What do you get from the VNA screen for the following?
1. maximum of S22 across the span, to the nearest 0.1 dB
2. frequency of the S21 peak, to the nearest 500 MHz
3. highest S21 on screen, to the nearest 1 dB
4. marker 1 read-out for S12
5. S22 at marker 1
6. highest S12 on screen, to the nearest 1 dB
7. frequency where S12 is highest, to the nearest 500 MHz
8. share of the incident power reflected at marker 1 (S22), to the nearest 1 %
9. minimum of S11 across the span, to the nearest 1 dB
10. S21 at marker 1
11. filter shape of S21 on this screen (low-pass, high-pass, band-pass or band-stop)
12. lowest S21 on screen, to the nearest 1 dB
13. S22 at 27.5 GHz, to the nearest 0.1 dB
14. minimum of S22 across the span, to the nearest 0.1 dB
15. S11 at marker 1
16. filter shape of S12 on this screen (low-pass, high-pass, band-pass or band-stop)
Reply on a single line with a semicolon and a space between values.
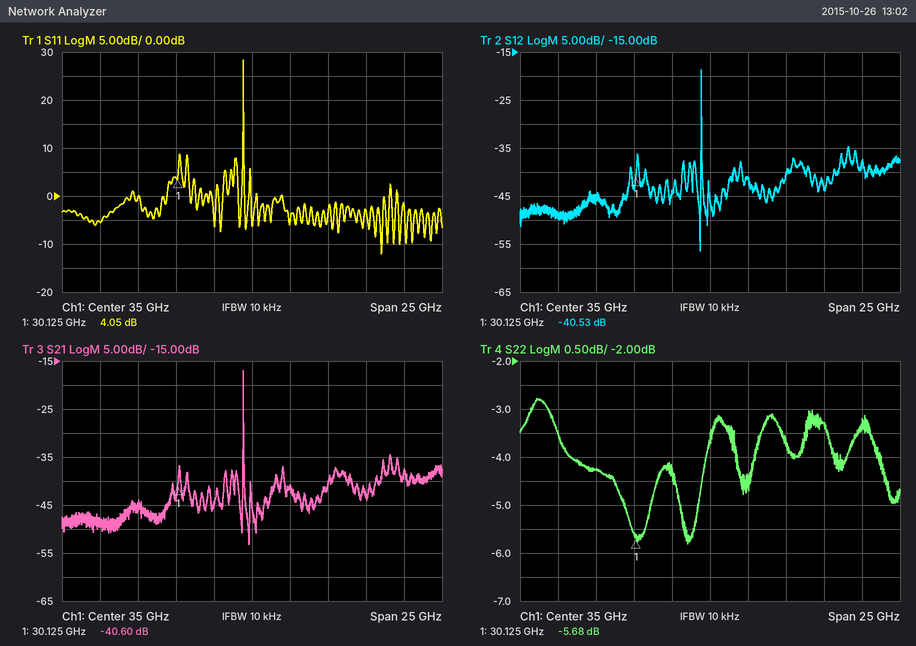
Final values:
-2.8 dB; 34.5 GHz; -17 dB; -40.53 dB; -5.68 dB; -19 dB; 34.5 GHz; 27 %; -12 dB; -40.60 dB; band-pass; -53 dB; -4.3 dB; -5.8 dB; 4.05 dB; band-pass
